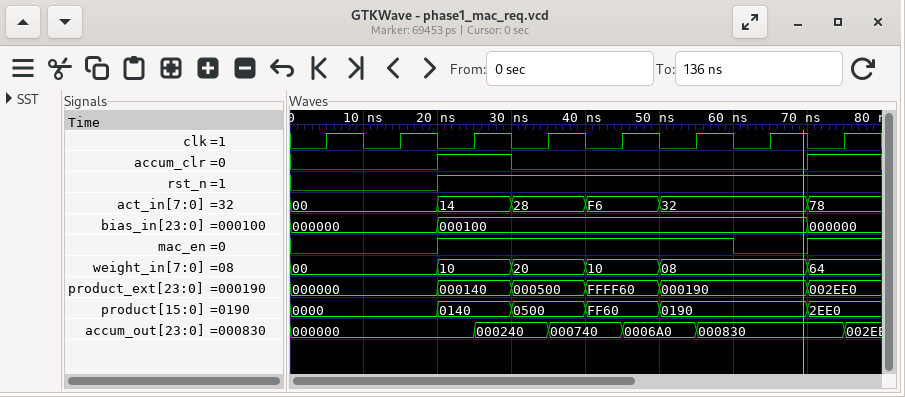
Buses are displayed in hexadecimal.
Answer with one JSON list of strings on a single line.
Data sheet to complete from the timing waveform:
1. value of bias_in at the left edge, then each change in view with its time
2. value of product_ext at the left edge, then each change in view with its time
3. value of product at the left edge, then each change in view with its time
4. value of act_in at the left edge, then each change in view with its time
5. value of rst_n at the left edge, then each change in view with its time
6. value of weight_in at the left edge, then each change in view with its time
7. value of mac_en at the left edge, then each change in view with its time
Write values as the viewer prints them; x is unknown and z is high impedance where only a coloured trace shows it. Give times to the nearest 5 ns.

["000000, 000100 at 20 ns, 000000 at 70 ns", "000000, 000140 at 20 ns, 000500 at 30 ns, FFFF60 at 40 ns, 000190 at 50 ns, 002EE0 at 70 ns", "0000, 0140 at 20 ns, 0500 at 30 ns, FF60 at 40 ns, 0190 at 50 ns, 2EE0 at 70 ns", "00, 14 at 20 ns, 28 at 30 ns, F6 at 40 ns, 32 at 50 ns, 78 at 70 ns", "0, 1 at 20 ns", "00, 10 at 20 ns, 20 at 30 ns, 10 at 40 ns, 08 at 50 ns, 64 at 70 ns", "0, 1 at 20 ns, 0 at 60 ns, 1 at 70 ns"]
